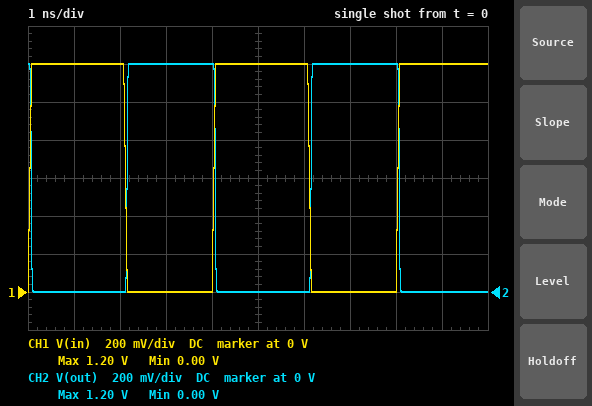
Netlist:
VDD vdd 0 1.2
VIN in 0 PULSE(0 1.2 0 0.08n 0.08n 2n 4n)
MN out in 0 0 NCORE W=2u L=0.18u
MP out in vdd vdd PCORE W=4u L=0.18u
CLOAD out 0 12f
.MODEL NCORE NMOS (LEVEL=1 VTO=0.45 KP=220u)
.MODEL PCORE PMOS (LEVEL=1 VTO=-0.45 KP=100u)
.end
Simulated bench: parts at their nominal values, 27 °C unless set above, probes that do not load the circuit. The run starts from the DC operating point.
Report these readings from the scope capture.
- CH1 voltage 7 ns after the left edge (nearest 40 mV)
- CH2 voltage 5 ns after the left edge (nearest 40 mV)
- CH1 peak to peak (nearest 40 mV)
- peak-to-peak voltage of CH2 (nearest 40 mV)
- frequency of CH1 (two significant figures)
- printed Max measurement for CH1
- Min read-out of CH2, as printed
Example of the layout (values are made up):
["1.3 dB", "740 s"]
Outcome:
["0 V", "0 V", "1.20 V", "1.20 V", "250 MHz", "1.20 V", "0.00 V"]
